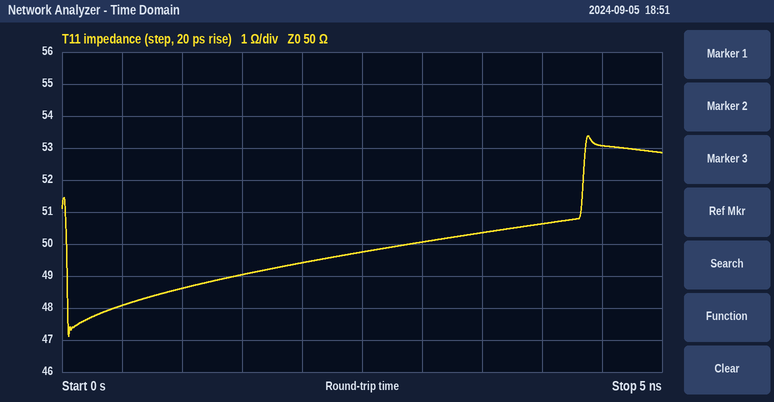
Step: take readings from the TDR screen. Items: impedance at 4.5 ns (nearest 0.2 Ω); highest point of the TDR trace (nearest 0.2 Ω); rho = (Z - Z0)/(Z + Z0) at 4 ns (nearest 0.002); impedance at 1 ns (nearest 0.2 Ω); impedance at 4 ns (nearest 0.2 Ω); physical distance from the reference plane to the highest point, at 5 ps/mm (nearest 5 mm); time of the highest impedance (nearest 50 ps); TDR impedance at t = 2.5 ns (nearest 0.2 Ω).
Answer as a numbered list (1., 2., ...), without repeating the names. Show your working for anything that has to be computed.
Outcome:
1. 53.0 Ω
2. 53.4 Ω
3. (50.6 − 50)/(50.6 + 50) ≈ +0.006
4. 48.6 Ω
5. 50.6 Ω
6. 4.40 ns / 2 / 5 ps/mm ≈ 440 mm
7. 4.40 ns
8. 49.8 Ω
